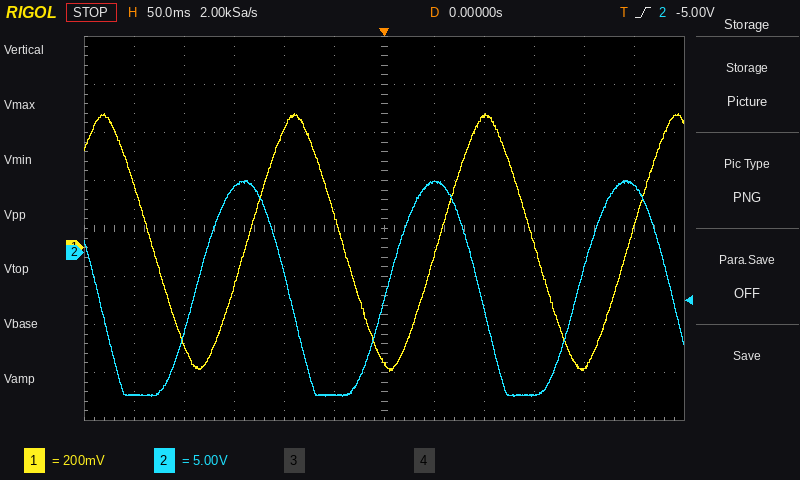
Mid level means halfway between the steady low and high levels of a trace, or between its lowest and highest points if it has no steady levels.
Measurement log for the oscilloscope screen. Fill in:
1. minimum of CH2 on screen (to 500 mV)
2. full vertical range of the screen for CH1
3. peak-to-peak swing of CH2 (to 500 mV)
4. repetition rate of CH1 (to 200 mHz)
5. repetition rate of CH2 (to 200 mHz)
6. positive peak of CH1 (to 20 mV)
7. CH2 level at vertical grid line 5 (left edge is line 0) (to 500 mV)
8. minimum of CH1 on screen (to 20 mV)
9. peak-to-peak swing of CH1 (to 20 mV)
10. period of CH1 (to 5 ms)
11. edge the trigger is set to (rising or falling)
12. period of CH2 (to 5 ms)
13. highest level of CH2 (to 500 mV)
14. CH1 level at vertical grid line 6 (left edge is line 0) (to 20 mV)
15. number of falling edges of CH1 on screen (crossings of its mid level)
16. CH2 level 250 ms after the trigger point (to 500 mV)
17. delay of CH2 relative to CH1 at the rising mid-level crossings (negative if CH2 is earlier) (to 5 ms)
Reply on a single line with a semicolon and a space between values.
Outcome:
-15.0 V; 1.6 V; 22.5 V; 5.2 Hz; 5.2 Hz; 560 mV; -15.0 V; -520 mV; 1.08 V; 190 ms; rising; 190 ms; 7.5 V; -480 mV; 3; 7.0 V; -50 ms
